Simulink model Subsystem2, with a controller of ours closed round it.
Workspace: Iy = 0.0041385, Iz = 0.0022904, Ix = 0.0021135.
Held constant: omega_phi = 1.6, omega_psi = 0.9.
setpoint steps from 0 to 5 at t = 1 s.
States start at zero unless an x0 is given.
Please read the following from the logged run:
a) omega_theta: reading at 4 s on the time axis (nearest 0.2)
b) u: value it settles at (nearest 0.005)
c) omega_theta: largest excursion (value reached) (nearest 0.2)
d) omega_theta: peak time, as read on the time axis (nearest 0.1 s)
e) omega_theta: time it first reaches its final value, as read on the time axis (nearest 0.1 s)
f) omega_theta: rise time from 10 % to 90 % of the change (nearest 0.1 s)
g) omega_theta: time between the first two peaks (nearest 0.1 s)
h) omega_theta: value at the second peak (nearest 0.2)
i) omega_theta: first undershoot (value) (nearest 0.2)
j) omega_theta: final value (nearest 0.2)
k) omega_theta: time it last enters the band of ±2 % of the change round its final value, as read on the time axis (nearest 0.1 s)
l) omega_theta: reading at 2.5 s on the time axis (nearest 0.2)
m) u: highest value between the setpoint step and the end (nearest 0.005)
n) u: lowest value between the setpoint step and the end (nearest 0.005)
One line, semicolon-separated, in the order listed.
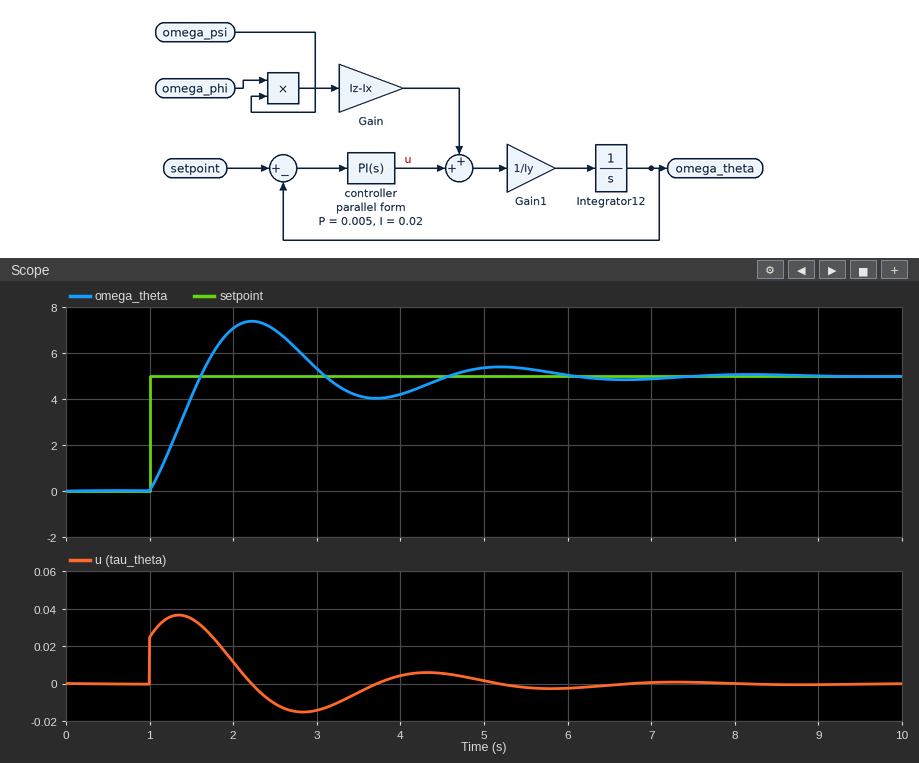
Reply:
4.2; 0.000; 7.4; 2.2 s; 1.6 s; 0.5 s; 3.0 s; 5.4; 4.0; 5.0; 7.1 s; 7.0; 0.035; -0.015
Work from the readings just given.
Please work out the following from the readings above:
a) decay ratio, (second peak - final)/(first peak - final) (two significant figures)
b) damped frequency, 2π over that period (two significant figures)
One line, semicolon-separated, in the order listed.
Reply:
0.17; 2.1 rad/s
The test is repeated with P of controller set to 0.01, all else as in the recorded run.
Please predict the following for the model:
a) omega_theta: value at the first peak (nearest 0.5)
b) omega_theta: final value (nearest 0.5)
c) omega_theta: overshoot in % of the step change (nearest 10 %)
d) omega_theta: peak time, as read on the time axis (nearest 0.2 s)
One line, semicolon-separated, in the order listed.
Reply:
6.5; 5.0; 30 %; 2.0 s
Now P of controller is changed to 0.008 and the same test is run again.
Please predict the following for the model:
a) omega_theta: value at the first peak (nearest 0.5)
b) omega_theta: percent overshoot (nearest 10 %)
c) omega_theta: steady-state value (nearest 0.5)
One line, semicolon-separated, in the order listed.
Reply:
6.5; 30 %; 5.0
